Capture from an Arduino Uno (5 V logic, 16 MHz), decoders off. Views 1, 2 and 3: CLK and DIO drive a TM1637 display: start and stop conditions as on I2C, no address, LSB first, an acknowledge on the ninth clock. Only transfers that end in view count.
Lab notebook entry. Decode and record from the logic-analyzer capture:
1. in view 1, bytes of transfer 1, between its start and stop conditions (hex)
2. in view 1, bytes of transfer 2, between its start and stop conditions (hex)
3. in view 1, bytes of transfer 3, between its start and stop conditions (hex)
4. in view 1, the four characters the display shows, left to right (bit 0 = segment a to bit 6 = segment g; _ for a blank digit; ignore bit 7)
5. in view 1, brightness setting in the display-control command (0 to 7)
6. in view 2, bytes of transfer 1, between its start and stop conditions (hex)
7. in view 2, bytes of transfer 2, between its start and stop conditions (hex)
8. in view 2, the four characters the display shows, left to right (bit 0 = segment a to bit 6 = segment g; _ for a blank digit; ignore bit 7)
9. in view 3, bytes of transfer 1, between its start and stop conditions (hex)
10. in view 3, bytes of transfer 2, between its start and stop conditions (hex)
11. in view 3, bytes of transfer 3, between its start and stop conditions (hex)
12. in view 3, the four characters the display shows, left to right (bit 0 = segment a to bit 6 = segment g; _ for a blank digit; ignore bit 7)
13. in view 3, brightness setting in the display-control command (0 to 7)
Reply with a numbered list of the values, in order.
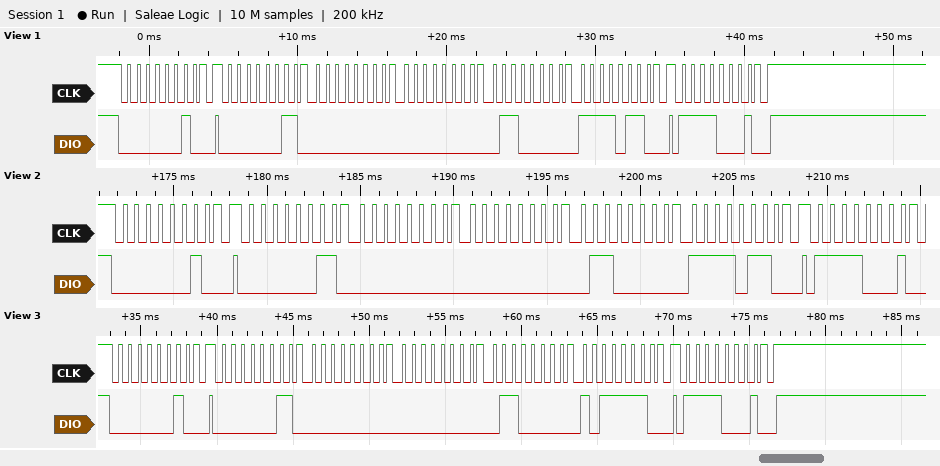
1. 40
2. C0 00 00 06 6F
3. 8F
4. __19
5. 7
6. 40
7. C0 00 00 06 6F
8. __19
9. 40
10. C0 00 00 06 7D
11. 8F
12. __16
13. 7
